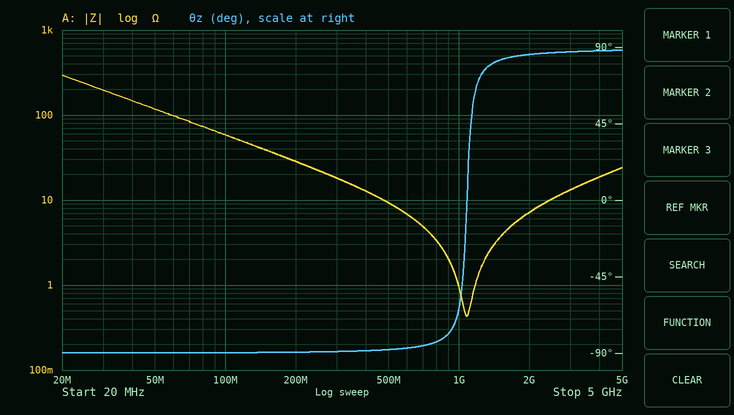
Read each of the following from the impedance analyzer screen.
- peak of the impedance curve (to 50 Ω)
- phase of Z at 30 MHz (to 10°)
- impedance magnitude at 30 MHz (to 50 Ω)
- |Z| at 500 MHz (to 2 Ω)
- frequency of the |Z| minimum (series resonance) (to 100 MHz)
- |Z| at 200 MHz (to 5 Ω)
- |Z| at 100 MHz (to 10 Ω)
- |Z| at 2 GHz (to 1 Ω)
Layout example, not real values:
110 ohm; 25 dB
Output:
300 Ω; -90°; 200 Ω; 10 Ω; 1.1 GHz; 30 Ω; 60 Ω; 7 Ω
